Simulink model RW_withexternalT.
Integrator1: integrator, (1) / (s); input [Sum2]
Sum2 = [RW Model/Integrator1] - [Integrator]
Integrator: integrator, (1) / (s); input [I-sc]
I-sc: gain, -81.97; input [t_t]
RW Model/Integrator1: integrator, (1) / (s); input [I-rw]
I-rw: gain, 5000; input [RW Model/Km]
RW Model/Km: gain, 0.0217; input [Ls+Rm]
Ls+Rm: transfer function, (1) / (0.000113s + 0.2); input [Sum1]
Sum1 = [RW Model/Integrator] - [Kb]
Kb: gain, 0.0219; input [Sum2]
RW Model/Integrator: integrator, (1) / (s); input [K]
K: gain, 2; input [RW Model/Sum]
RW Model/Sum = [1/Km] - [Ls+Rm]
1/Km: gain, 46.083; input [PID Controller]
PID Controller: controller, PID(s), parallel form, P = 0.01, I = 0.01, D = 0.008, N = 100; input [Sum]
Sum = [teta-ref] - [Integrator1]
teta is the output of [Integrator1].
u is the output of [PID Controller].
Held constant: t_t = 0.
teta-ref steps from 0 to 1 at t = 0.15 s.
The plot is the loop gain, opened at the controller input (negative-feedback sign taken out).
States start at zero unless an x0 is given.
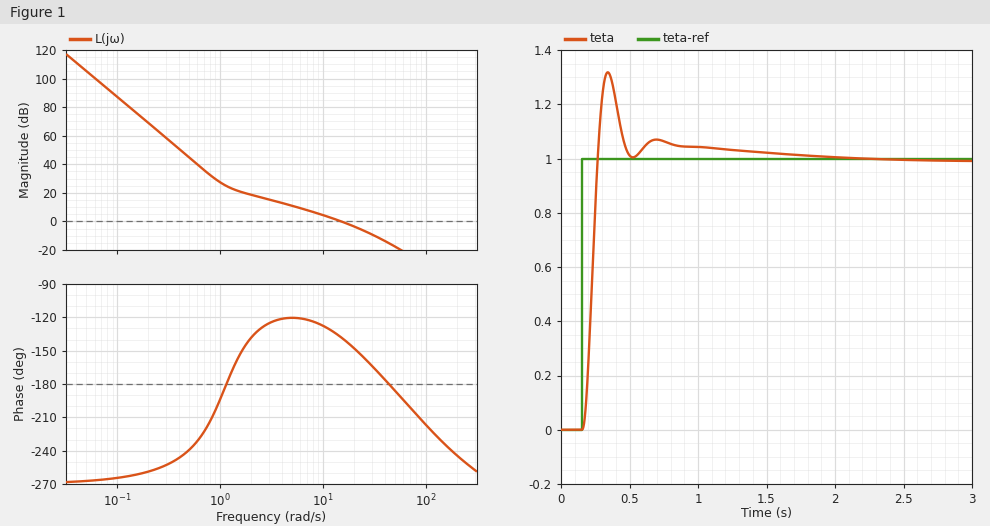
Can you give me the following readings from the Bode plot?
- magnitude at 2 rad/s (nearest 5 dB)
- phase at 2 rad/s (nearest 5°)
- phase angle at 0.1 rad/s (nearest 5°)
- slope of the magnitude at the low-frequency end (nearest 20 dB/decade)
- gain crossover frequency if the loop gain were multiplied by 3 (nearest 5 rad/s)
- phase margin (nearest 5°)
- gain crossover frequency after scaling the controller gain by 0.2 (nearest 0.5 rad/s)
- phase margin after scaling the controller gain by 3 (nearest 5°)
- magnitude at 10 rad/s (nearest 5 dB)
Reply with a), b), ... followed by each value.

a) 20 dB
b) -140°
c) -265°
d) -60 dB/decade
e) 30 rad/s
f) 40°
g) 3.5 rad/s
h) 15°
i) 5 dB
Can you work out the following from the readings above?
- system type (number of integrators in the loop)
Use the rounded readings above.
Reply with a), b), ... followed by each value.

a) 3
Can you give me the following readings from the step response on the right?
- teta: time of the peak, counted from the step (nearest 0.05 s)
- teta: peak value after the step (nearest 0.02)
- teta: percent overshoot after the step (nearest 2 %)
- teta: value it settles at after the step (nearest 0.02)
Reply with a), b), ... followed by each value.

a) 0.20 s
b) 1.32
c) 32 %
d) 1.00
